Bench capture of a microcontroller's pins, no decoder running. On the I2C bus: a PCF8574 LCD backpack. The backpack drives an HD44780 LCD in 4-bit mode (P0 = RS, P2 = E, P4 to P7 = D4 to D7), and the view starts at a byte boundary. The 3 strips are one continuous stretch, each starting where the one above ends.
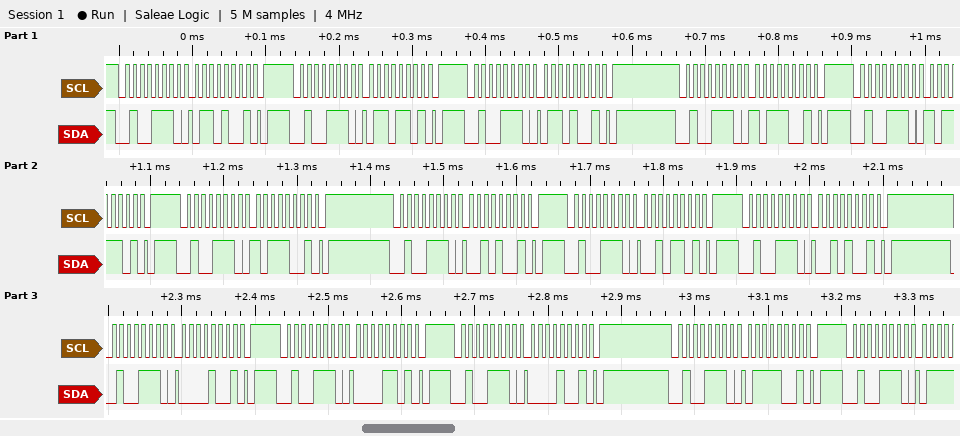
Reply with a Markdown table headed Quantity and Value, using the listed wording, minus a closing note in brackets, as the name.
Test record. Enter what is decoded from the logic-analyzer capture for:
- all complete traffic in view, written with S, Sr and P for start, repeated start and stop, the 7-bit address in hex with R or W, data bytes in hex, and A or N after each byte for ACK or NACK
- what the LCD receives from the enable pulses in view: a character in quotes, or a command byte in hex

| Quantity | Value |
|---|---|
| all complete traffic in view, written with S, Sr and P for start, repeated start and stop, the 7-bit address in hex with R or W, data bytes in hex, and A or N after each byte for ACK or NACK | S 27W A 69 A P S 27W A 6D A P S 27W A 69 A P S 27W A B9 A P S 27W A BD A P S 27W A B9 A P S 27W A 29 A P S 27W A 2D A P S 27W A 29 A P S 27W A 09 A P S 27W A 0D A P S 27W A 09 A P S 27W A 79 A P S 27W A |
| what the LCD receives from the enable pulses in view: a character in quotes, or a command byte in hex | 'k' ' ' |
